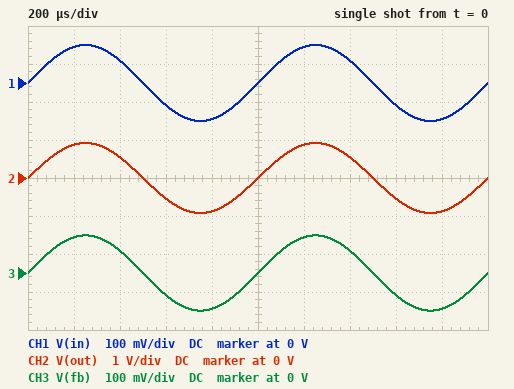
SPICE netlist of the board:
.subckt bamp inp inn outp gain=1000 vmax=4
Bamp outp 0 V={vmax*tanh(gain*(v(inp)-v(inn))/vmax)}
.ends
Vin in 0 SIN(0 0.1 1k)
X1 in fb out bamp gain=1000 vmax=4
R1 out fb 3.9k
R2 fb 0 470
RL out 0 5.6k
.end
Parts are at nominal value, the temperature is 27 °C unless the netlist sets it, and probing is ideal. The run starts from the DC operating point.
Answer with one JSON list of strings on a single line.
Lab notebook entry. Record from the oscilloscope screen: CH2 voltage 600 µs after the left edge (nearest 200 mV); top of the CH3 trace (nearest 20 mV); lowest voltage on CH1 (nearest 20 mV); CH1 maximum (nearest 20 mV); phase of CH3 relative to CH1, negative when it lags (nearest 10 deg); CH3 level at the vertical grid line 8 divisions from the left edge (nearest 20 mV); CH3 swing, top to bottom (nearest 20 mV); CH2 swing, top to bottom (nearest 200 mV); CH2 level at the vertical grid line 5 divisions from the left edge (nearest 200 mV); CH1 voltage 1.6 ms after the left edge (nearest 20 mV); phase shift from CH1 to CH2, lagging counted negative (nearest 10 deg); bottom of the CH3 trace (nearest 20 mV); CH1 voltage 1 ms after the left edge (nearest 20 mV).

["-600 mV", "100 mV", "-100 mV", "100 mV", "0 deg", "-60 mV", "200 mV", "1.8 V", "0 V", "-60 mV", "0 deg", "-100 mV", "0 V"]
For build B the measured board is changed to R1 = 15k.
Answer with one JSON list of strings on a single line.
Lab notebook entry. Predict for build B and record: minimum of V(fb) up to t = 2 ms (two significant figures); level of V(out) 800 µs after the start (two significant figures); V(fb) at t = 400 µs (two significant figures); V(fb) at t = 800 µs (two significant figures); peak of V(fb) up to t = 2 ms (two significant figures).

["-96 mV", "-3.0 V", "57 mV", "-91 mV", "96 mV"]
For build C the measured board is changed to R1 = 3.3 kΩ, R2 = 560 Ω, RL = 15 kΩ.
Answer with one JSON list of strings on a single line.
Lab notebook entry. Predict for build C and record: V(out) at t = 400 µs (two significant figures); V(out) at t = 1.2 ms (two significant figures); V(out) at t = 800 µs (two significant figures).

["400 mV", "650 mV", "-650 mV"]
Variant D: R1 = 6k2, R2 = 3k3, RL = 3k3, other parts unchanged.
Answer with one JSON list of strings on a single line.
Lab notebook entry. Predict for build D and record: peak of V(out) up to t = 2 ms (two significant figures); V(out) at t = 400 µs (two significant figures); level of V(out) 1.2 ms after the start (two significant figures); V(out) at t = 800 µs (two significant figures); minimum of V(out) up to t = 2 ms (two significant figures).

["290 mV", "170 mV", "270 mV", "-270 mV", "-290 mV"]
